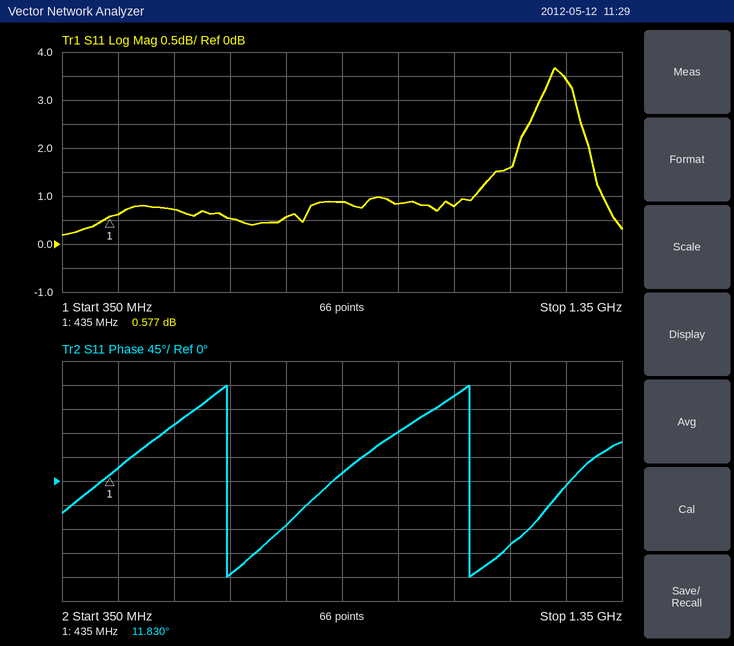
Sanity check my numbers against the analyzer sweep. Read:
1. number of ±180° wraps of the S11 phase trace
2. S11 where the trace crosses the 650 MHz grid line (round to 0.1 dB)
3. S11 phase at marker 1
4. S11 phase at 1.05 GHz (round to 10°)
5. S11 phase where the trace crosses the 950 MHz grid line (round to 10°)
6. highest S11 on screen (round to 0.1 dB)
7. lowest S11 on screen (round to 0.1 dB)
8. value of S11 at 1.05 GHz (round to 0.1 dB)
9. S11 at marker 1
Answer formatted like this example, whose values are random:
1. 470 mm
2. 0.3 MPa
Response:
1. 2
2. 0.5 dB
3. 11.830°
4. 160°
5. 90°
6. 3.7 dB
7. 0.2 dB
8. 0.8 dB
9. 0.577 dB
